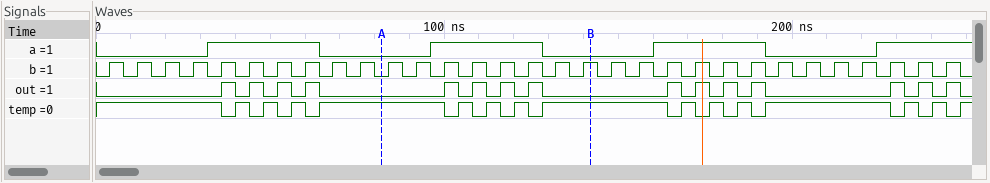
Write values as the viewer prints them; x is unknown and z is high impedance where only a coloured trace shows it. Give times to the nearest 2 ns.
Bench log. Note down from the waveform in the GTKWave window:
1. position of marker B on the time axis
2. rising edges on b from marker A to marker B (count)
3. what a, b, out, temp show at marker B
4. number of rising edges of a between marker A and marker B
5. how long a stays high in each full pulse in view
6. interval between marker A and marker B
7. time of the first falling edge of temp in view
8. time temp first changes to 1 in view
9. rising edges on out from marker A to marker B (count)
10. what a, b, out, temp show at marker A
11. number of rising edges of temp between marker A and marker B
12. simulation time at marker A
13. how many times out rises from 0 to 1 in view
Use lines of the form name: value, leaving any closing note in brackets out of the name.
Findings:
position of marker B on the time axis: 142 ns
rising edges on b from marker A to marker B: 8
what a, b, out, temp show at marker B: a=0, b=1, out=0, temp=1
number of rising edges of a between marker A and marker B: 1
how long a stays high in each full pulse in view: 32 ns, 32 ns, 32 ns
interval between marker A and marker B: 60 ns
time of the first falling edge of temp in view: 36 ns
time temp first changes to 1 in view: 40 ns
rising edges on out from marker A to marker B: 4
what a, b, out, temp show at marker A: a=0, b=0, out=0, temp=1
number of rising edges of temp between marker A and marker B: 4
simulation time at marker A: 82 ns
how many times out rises from 0 to 1 in view: 15
